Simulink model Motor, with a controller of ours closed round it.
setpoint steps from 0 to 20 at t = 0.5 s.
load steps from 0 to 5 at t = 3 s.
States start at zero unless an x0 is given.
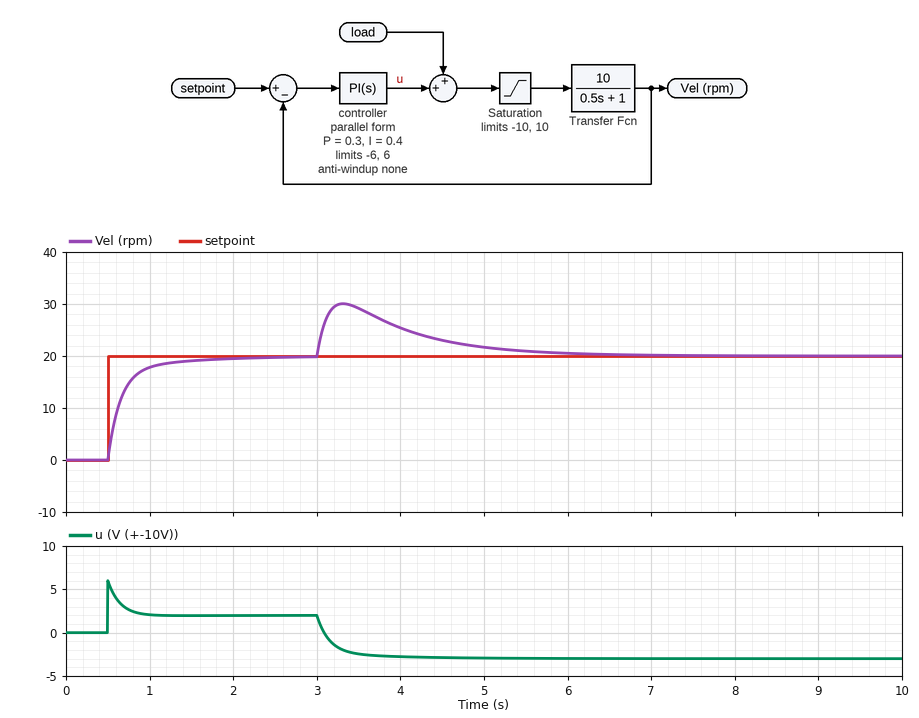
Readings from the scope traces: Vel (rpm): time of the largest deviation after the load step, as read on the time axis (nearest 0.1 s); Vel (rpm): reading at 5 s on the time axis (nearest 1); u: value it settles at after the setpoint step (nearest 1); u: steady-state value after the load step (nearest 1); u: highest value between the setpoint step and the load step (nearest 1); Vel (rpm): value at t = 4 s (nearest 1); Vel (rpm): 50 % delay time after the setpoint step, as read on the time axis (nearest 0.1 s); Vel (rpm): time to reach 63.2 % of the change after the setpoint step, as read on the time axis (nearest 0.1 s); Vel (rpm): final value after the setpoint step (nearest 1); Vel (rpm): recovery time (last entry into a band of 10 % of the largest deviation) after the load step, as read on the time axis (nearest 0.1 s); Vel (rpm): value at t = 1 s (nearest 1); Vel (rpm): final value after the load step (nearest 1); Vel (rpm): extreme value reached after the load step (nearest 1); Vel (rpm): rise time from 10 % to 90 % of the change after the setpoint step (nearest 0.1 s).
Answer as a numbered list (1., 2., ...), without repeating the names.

1. 3.3 s
2. 22
3. 2
4. -3
5. 6
6. 25
7. 0.6 s
8. 0.7 s
9. 20
10. 5.4 s
11. 18
12. 20
13. 30
14. 0.5 s
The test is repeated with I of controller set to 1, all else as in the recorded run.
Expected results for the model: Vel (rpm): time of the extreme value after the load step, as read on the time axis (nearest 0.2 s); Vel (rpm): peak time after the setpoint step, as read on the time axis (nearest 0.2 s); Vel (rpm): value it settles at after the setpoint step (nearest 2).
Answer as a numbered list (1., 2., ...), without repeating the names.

1. 3.2 s
2. 1.2 s
3. 20
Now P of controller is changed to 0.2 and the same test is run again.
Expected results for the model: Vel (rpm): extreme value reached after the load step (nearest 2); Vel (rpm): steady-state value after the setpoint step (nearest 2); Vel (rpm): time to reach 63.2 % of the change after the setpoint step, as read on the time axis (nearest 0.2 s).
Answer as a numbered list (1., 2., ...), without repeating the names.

1. 32
2. 20
3. 0.8 s
